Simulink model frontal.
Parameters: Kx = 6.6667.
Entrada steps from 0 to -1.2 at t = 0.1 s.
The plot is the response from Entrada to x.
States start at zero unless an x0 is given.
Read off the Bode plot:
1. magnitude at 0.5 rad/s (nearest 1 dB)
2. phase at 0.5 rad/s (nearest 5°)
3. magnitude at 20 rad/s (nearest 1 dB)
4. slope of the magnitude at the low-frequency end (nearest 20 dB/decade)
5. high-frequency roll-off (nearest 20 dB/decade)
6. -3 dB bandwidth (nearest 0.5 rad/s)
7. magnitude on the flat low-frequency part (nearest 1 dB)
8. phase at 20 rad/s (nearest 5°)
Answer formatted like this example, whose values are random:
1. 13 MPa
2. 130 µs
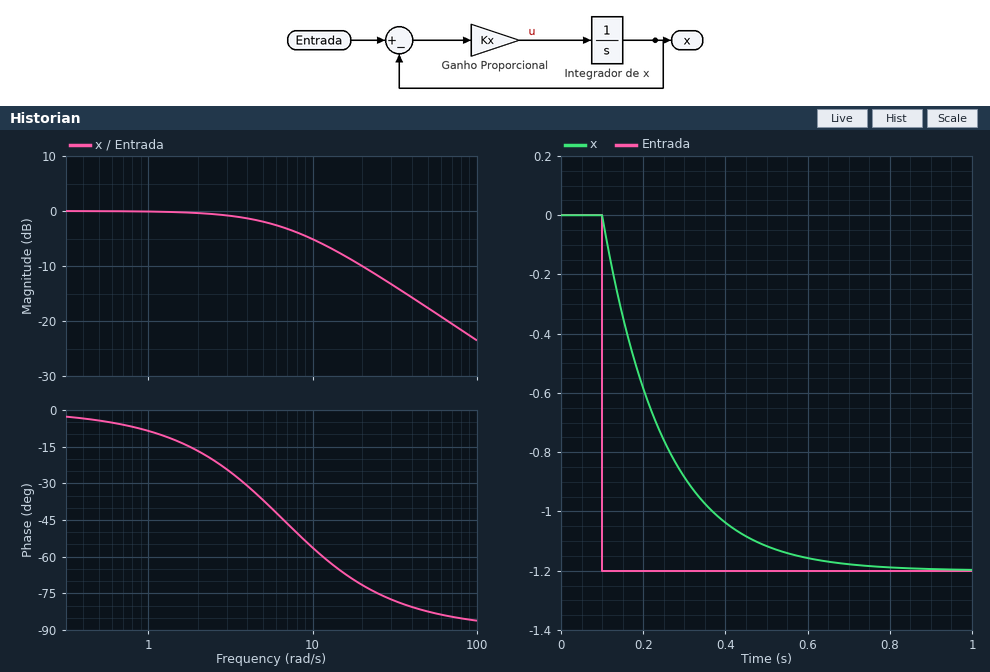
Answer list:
1. 0 dB
2. -5°
3. -10 dB
4. 0 dB/decade
5. -20 dB/decade
6. 6.5 rad/s
7. 0 dB
8. -70°
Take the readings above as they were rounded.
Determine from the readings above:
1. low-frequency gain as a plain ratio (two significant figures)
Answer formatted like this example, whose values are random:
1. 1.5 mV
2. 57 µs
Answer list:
1. 1.0
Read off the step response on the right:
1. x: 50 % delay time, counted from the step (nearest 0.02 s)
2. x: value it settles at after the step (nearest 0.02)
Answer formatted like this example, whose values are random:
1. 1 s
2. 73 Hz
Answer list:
1. 0.10 s
2. -1.20
